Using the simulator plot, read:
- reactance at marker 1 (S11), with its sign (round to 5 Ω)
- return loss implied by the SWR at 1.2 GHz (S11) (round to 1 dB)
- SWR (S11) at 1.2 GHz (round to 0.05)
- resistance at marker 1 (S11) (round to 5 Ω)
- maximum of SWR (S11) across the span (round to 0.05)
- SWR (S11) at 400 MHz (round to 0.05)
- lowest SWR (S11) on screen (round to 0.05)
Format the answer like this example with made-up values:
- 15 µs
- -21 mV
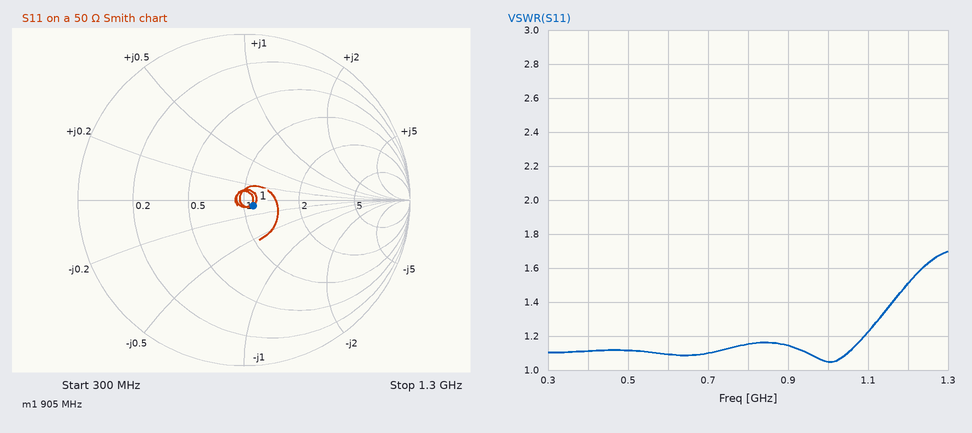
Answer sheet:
- -5 Ω
- 14 dB
- 1.50
- 55 Ω
- 1.70
- 1.10
- 1.05
